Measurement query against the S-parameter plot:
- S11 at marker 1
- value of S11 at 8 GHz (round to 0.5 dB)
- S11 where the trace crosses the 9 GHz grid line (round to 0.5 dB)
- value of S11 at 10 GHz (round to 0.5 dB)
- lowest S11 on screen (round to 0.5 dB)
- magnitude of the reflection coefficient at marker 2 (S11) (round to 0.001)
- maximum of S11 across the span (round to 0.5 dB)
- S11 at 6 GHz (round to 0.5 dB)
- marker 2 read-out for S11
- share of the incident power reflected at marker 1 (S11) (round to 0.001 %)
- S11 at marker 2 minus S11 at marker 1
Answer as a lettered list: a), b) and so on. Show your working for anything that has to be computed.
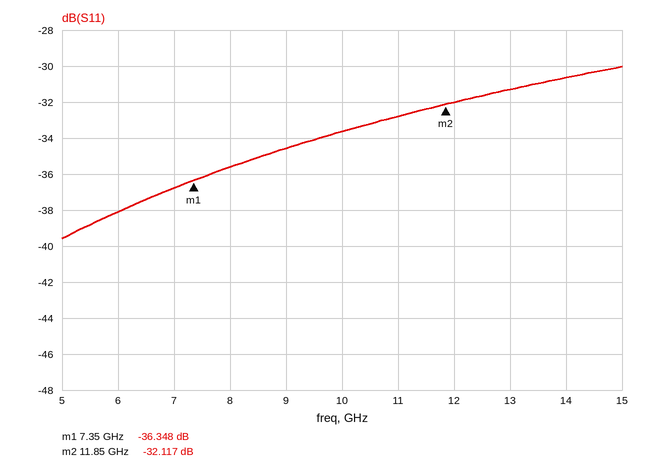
a) -36.348 dB
b) -35.5 dB
c) -34.5 dB
d) -33.5 dB
e) -39.5 dB
f) 10^(-32.117/20) ≈ 0.025
g) -30.0 dB
h) -38.0 dB
i) -32.117 dB
j) 10^(-36.348/10) ≈ 0.023 %
k) -32.117 − (-36.348) = 4.231 dB
